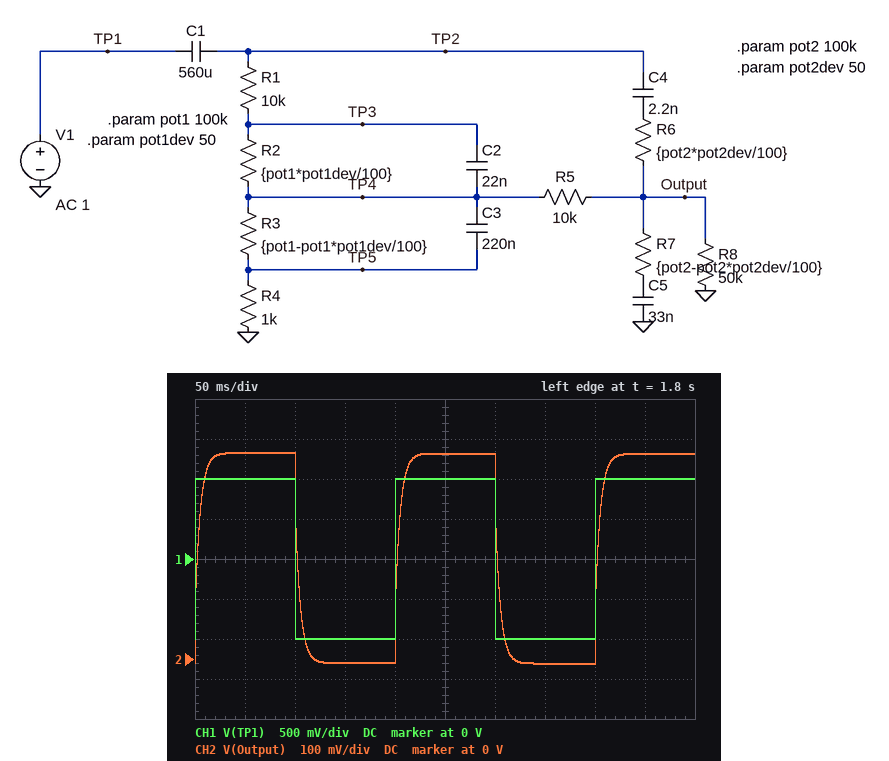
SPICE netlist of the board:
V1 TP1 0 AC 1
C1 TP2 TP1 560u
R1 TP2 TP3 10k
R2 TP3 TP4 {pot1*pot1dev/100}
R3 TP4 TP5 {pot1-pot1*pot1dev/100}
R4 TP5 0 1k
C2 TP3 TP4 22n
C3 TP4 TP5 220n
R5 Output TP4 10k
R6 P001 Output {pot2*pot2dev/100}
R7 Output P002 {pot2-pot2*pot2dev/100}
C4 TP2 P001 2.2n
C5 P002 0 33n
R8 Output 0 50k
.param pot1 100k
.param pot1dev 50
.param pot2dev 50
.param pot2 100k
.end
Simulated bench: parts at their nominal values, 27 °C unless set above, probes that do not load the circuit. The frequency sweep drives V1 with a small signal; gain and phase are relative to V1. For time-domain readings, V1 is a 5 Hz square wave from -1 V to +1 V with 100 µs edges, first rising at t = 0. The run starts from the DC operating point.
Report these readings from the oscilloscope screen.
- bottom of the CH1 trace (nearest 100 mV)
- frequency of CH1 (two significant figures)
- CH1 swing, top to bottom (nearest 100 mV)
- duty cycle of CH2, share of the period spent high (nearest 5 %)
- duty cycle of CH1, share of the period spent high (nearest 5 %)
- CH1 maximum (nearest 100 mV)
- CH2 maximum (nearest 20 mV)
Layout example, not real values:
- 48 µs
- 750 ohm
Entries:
- -1.0 V
- 5.0 Hz
- 2.0 V
- 50 %
- 50 %
- 1.0 V
- 520 mV
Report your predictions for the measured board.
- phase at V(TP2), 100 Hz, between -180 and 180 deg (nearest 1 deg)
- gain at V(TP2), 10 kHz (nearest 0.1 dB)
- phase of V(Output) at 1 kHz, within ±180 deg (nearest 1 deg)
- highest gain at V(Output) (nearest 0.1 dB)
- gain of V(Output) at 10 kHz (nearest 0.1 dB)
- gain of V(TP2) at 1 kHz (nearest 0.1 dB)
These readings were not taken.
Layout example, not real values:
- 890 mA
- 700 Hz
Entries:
- 0 deg
- 0 dB
- 26 deg
- -11.6 dB
- -14.6 dB
- 0 dB
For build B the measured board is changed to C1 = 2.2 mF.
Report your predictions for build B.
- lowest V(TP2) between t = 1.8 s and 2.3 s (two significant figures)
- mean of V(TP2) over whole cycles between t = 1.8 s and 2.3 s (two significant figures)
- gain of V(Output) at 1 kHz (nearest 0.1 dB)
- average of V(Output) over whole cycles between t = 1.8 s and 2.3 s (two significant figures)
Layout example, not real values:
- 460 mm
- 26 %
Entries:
- -11 mV
- 990 mV
- -18.1 dB
- 260 mV
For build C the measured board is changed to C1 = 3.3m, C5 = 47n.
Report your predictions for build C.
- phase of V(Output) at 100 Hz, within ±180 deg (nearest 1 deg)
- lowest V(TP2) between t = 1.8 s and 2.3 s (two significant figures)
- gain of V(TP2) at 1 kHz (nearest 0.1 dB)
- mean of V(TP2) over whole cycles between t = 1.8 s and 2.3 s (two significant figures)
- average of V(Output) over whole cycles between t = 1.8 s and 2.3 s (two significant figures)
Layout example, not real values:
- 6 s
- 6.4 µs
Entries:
- -29 deg
- -7.6 mV
- 0 dB
- 990 mV
- 260 mV
